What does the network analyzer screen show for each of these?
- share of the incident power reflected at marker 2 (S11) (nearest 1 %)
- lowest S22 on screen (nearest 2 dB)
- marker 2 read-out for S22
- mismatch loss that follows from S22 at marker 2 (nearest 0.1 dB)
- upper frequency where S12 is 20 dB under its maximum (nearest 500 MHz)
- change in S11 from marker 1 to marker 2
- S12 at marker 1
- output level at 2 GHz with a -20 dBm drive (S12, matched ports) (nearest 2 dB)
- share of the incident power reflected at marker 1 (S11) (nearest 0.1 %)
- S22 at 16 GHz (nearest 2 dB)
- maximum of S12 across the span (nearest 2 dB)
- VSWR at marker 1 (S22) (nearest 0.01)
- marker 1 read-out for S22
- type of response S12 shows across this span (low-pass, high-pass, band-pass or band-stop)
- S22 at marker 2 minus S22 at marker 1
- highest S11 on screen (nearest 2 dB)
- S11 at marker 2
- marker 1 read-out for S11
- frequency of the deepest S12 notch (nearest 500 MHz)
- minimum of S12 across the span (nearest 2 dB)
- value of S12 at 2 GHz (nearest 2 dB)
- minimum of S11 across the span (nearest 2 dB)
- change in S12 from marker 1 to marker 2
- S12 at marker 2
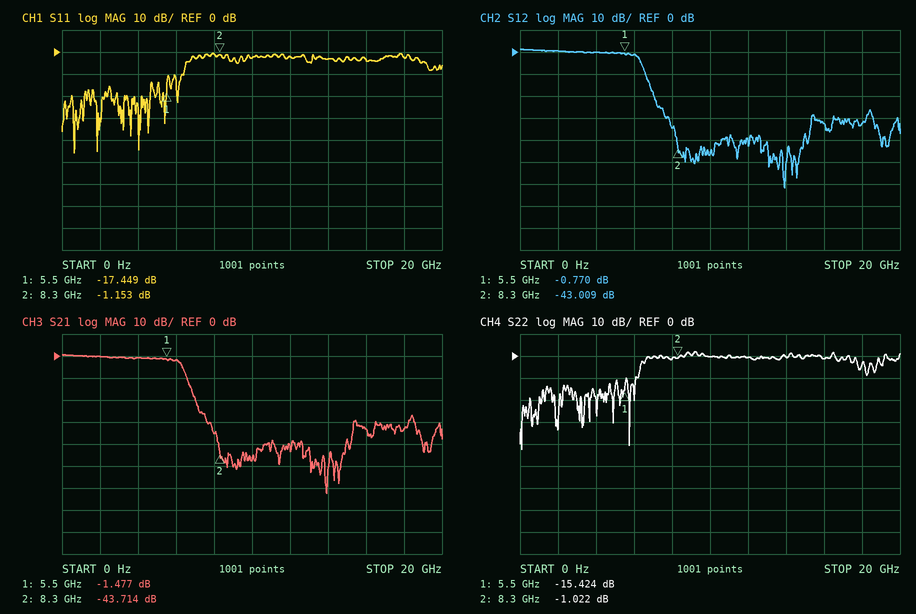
77 %
-42 dB
-1.022 dB
6.8 dB
7.0 GHz
16.296 dB
-0.770 dB
-20 dBm
1.8 %
-2 dB
2 dB
1.41
-15.424 dB
low-pass
14.402 dB
0 dB
-1.153 dB
-17.449 dB
14.0 GHz
-62 dB
0 dB
-46 dB
-42.239 dB
-43.009 dB
